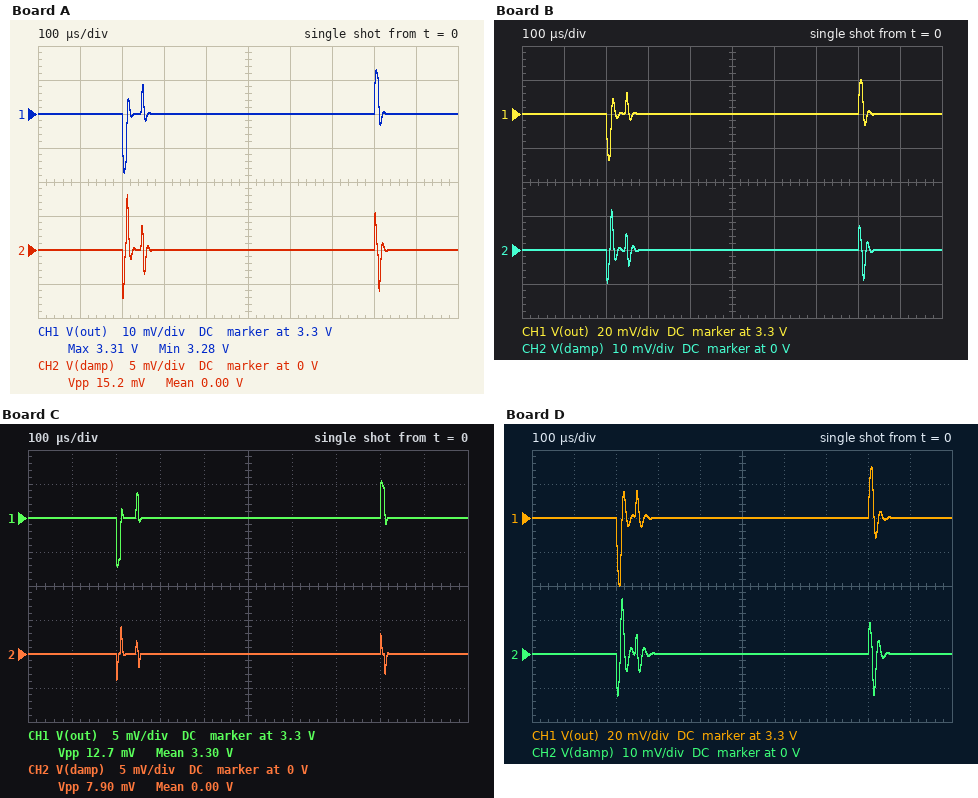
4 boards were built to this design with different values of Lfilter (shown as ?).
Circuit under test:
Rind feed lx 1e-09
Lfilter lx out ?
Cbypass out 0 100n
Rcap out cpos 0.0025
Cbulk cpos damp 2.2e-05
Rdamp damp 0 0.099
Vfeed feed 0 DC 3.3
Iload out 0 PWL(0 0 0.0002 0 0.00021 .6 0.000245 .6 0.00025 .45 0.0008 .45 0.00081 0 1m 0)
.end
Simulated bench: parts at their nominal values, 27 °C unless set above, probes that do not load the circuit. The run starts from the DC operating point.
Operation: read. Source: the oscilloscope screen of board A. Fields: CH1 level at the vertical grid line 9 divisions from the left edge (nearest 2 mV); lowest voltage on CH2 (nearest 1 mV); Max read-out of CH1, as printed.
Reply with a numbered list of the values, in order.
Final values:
1. 3.300 V
2. -7 mV
3. 3.31 V
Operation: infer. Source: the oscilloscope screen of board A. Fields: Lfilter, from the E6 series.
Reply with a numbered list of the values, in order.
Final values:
1. 220 nH
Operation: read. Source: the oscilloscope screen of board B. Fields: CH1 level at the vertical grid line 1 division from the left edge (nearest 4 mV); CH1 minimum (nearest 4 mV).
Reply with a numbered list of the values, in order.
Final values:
1. 3.300 V
2. 3.272 V
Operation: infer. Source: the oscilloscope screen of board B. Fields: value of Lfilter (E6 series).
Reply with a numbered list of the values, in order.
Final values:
1. 330 nH
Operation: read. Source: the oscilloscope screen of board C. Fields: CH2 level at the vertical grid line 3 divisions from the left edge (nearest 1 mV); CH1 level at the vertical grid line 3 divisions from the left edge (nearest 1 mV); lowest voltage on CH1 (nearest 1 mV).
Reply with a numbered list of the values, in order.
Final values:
1. 0 V
2. 3.300 V
3. 3.293 V
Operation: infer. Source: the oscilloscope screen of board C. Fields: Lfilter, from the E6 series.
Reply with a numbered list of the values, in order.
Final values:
1. 100 nH
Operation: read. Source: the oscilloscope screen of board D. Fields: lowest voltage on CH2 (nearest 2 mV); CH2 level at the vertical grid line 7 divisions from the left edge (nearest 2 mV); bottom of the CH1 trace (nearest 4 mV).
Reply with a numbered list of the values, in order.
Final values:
1. -12 mV
2. 0 V
3. 3.260 V
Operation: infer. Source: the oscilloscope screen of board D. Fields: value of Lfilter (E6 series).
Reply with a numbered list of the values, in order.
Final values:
1. 470 nH
